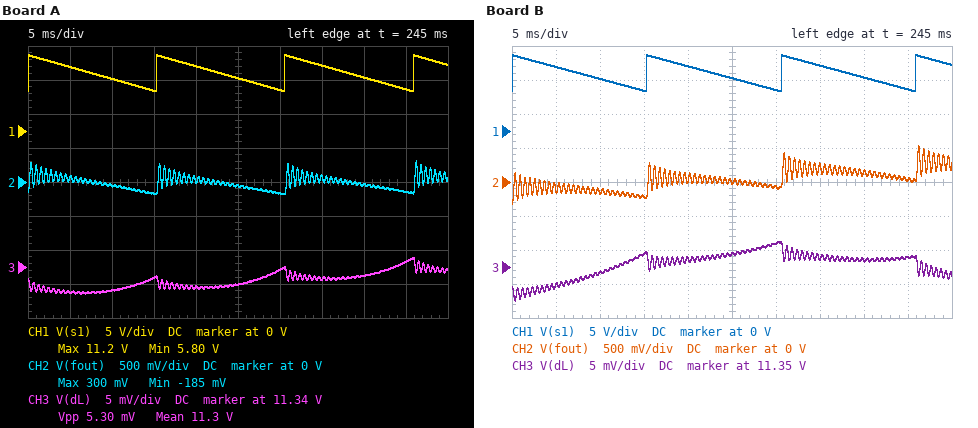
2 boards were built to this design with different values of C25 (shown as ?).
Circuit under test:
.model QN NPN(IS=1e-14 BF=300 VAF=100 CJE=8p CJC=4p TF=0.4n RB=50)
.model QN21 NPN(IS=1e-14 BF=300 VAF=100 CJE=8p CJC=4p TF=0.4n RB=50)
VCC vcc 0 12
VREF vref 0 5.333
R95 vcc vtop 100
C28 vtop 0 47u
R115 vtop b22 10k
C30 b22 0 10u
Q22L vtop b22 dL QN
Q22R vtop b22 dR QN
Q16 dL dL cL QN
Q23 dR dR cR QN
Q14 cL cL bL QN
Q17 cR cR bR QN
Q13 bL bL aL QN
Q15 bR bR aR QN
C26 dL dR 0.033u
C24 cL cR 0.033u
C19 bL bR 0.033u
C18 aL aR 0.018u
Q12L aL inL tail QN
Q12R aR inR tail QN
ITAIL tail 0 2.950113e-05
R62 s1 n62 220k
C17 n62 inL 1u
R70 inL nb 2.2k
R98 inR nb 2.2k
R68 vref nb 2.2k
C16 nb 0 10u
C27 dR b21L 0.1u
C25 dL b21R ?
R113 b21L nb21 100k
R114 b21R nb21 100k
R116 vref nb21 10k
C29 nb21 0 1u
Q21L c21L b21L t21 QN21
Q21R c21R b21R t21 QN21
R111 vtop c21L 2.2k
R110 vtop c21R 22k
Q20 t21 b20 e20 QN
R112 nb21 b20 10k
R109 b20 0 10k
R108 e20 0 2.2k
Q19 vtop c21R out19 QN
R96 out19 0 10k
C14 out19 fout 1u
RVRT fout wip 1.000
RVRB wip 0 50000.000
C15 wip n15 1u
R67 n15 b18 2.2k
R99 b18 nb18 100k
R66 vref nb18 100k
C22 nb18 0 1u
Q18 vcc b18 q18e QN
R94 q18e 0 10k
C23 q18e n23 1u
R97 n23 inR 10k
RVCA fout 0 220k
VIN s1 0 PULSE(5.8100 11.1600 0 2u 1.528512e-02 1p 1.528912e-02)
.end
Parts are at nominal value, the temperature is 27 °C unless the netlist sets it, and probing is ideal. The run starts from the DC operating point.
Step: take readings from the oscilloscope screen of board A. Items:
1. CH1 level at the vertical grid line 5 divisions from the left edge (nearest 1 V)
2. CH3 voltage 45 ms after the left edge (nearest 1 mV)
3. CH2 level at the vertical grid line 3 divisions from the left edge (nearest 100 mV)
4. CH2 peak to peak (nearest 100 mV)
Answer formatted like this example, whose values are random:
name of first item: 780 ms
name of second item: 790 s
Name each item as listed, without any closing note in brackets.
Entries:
CH1 level at the vertical grid line 5 divisions from the left edge: 8 V
CH3 voltage 45 ms after the left edge: 11.341 V
CH2 level at the vertical grid line 3 divisions from the left edge: -200 mV
CH2 peak to peak: 500 mV
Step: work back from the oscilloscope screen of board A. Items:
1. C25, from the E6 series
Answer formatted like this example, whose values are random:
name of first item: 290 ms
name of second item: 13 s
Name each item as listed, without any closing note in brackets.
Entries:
C25, from the E6 series: 47 nF
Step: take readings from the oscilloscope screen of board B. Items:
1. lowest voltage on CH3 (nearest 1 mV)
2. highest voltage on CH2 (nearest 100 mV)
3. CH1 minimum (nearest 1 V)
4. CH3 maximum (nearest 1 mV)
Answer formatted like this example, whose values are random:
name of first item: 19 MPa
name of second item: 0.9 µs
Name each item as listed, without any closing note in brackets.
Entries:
lowest voltage on CH3: 11.340 V
highest voltage on CH2: 500 mV
CH1 minimum: 6 V
CH3 maximum: 11.349 V
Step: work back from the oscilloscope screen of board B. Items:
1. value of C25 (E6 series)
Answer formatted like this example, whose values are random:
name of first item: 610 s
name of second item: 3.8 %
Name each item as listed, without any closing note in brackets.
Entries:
value of C25: 330 nF
